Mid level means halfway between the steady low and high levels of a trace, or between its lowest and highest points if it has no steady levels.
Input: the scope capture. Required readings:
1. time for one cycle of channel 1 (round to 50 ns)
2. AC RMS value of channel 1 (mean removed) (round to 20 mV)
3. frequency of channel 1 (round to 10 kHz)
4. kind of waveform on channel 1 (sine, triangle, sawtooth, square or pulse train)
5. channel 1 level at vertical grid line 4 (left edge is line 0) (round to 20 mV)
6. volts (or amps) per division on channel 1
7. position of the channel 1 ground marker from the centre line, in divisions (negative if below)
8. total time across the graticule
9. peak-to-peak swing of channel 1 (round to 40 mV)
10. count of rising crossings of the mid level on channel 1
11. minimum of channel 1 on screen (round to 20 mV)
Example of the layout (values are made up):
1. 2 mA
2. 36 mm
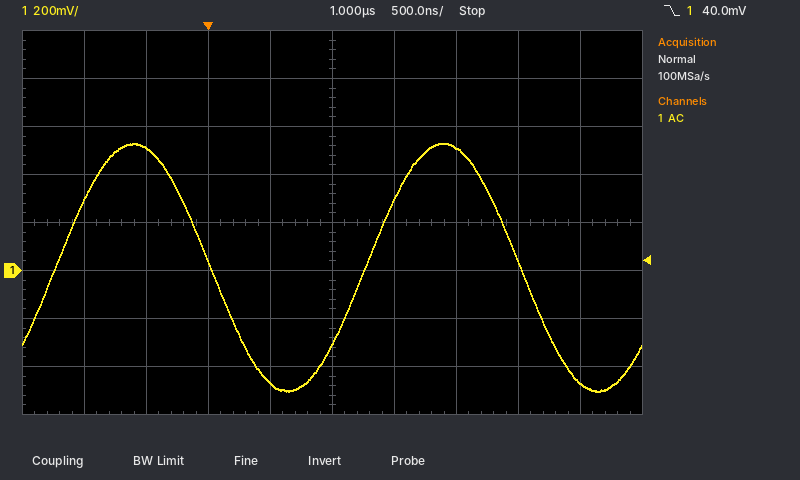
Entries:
1. 2.50 µs
2. 360 mV
3. 400 kHz
4. sine
5. -460 mV
6. 200 mV
7. -1.0 div
8. 5 µs
9. 1.04 V
10. 2
11. -500 mV
